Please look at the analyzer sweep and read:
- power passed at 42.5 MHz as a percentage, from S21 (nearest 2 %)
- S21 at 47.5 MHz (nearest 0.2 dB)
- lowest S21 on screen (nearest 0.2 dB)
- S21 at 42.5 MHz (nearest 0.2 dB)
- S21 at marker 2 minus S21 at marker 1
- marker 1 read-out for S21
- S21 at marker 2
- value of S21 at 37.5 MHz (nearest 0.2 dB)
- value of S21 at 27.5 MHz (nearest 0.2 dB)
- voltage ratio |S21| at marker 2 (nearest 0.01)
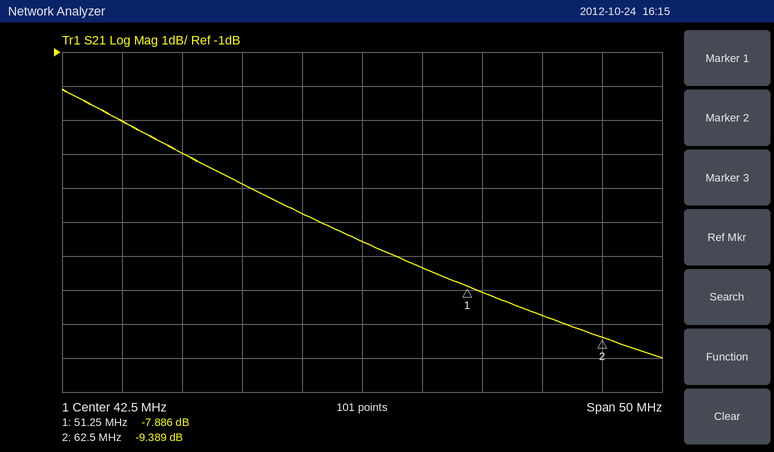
22 %
-7.4 dB
-10.0 dB
-6.6 dB
-1.503 dB
-7.886 dB
-9.389 dB
-5.8 dB
-4.0 dB
0.34
